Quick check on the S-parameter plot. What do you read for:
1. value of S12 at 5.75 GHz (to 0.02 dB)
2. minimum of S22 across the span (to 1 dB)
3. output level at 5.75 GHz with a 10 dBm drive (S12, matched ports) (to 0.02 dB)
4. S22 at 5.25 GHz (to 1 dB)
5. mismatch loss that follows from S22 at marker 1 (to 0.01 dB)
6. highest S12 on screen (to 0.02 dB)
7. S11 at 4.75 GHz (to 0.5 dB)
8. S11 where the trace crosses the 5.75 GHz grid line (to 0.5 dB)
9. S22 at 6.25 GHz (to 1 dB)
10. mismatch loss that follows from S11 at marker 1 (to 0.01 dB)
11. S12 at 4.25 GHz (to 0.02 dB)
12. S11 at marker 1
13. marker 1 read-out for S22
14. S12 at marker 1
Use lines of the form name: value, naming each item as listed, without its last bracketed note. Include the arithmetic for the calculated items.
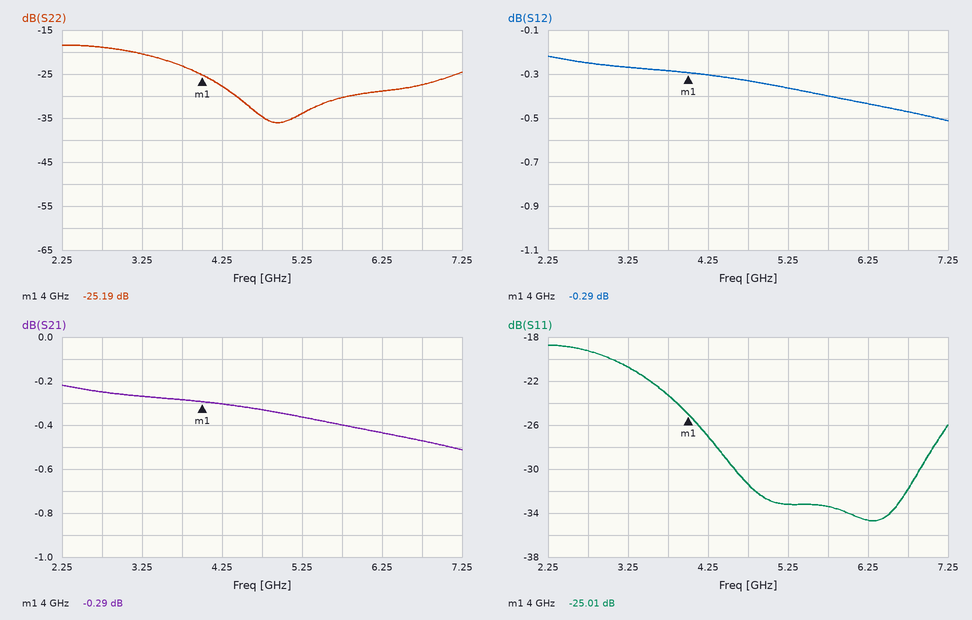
value of S12 at 5.75 GHz: -0.40 dB
minimum of S22 across the span: -36 dB
output level at 5.75 GHz with a 10 dBm drive (S12, matched ports): 10 dBm + (-0.40 dB) = 9.60 dBm
S22 at 5.25 GHz: -34 dB
mismatch loss that follows from S22 at marker 1: −10 log10(1 − 10^(-25.19/10)) ≈ 0.01 dB
highest S12 on screen: -0.22 dB
S11 at 4.75 GHz: -31.5 dB
S11 where the trace crosses the 5.75 GHz grid line: -33.5 dB
S22 at 6.25 GHz: -29 dB
mismatch loss that follows from S11 at marker 1: −10 log10(1 − 10^(-25.01/10)) ≈ 0.01 dB
S12 at 4.25 GHz: -0.30 dB
S11 at marker 1: -25.01 dB
marker 1 read-out for S22: -25.19 dB
S12 at marker 1: -0.29 dB
